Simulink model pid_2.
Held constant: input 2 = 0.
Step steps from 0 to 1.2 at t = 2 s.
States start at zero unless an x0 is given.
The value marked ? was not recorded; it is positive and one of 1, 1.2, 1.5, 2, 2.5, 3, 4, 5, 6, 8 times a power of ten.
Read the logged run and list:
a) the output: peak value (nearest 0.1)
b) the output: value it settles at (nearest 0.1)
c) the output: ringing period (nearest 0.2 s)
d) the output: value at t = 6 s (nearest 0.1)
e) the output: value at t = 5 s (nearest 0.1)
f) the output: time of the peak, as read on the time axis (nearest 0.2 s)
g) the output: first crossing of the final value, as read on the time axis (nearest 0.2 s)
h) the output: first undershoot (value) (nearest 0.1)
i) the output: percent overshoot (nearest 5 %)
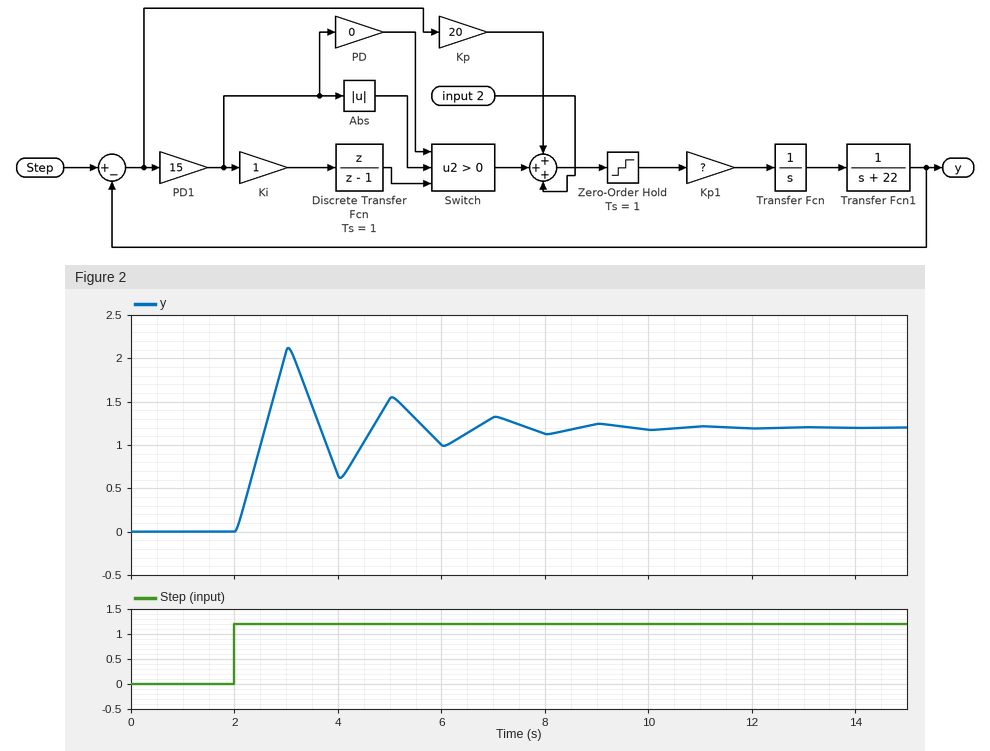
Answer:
2.1
1.2
2.0 s
1.0
1.5
3.0 s
2.6 s
0.6
75 %
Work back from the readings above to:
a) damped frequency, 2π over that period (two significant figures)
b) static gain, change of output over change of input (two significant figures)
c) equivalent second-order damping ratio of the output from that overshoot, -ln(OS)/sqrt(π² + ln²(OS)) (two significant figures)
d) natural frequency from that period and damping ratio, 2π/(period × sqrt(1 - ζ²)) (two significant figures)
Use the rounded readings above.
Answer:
3.1 rad/s
1.0
0.091
3.2 rad/s
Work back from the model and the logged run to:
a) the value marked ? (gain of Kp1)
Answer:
2
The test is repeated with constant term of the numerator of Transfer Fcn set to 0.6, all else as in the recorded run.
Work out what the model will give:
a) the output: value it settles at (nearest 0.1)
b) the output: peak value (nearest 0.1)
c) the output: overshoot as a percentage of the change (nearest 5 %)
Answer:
1.2
1.3
10 %
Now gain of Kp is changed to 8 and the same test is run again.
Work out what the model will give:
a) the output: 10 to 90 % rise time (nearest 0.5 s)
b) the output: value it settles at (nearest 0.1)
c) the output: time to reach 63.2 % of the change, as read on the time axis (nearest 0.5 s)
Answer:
1.5 s
1.2
3.0 s
